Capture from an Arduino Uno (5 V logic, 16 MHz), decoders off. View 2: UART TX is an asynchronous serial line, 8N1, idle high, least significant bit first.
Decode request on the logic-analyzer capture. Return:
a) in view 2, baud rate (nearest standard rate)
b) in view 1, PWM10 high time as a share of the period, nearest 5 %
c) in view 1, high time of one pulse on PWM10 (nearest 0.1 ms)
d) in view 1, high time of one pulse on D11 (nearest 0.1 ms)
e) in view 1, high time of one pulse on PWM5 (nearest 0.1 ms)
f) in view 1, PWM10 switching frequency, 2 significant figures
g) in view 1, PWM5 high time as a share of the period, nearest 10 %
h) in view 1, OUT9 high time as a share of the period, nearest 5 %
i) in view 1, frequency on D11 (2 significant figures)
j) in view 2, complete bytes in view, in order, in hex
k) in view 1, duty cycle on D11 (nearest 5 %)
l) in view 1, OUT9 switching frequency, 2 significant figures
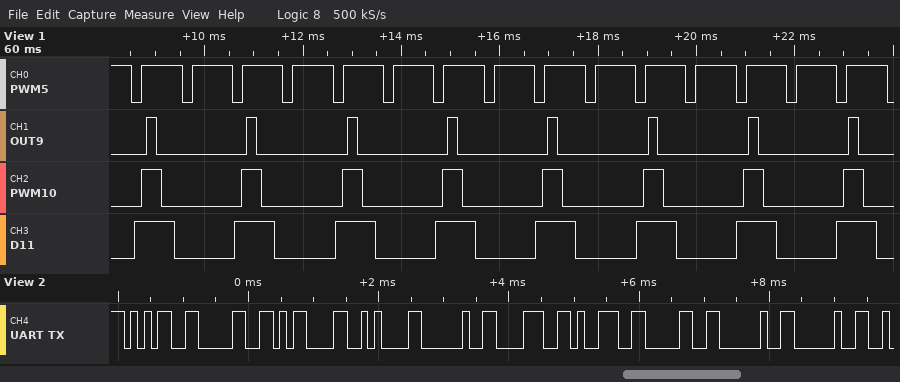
9600 baud
20 %
0.4 ms
0.8 ms
0.8 ms
490 Hz
80 %
10 %
490 Hz
0x35 0x30 0x0D 0x0A 0x20 0x38 0x39 0x30 0x20 0x20
40 %
490 Hz
